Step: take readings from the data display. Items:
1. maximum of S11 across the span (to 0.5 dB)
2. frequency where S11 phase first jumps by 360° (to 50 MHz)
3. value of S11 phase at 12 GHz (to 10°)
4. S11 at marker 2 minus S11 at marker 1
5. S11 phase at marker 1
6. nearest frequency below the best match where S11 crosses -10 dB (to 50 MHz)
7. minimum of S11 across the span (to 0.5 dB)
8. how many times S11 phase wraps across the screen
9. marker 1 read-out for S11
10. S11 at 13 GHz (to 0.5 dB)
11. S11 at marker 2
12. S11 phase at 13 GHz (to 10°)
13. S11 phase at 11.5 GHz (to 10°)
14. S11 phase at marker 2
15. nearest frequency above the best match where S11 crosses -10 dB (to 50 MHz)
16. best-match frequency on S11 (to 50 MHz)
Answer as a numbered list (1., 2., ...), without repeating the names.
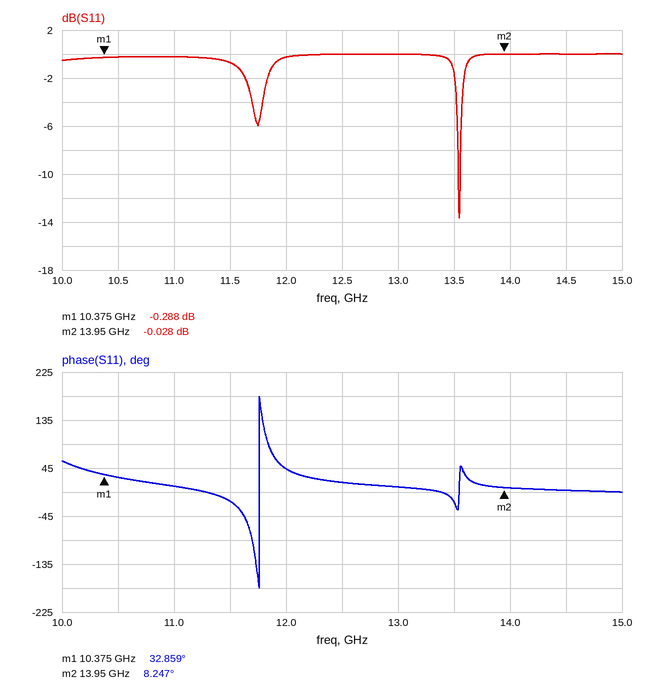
1. 0.0 dB
2. 11.75 GHz
3. 40°
4. 0.260 dB
5. 32.859°
6. 13.55 GHz
7. -13.5 dB
8. 1
9. -0.288 dB
10. 0.0 dB
11. -0.028 dB
12. 10°
13. -20°
14. 8.247°
15. 13.55 GHz
16. 13.55 GHz
